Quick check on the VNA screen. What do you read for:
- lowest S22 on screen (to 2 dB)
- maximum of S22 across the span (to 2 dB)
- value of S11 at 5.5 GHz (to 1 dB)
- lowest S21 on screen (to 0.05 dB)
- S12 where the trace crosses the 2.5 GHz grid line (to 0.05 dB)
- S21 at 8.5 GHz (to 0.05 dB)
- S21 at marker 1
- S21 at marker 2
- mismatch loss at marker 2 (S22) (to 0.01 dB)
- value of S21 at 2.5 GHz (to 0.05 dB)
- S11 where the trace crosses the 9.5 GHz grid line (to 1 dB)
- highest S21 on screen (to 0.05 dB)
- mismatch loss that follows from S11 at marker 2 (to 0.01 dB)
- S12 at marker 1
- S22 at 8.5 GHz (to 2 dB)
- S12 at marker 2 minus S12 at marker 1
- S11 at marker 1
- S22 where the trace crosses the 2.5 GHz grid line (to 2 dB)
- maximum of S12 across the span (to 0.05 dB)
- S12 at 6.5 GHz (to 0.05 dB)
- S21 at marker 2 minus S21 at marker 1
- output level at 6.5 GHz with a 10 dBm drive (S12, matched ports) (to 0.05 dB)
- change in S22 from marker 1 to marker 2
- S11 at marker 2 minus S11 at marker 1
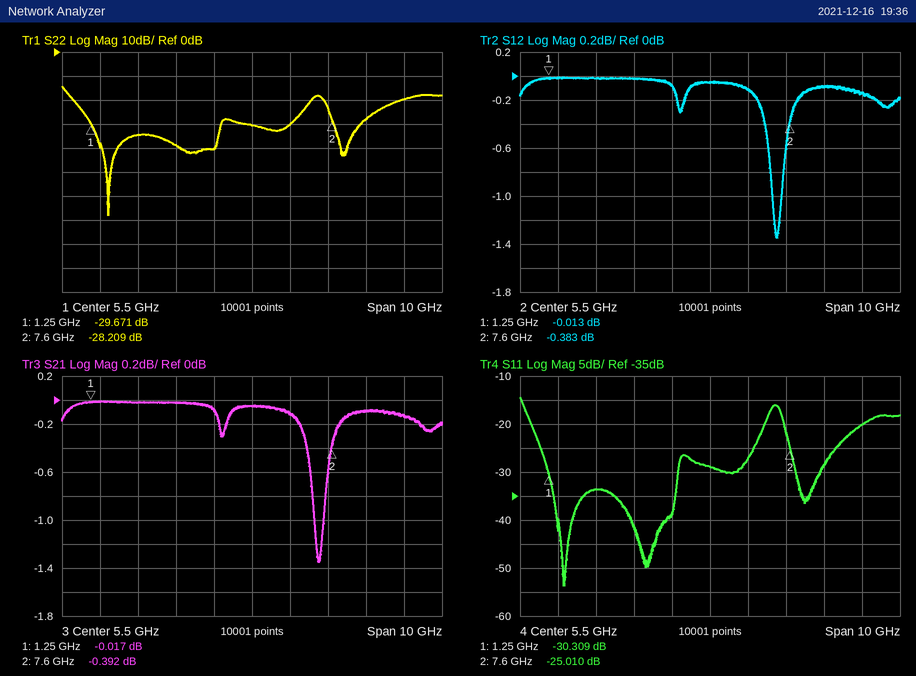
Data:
-68 dB
-14 dB
-29 dB
-1.35 dB
0.00 dB
-0.10 dB
-0.017 dB
-0.392 dB
0.01 dB
0.00 dB
-20 dB
0.00 dB
0.01 dB
-0.013 dB
-28 dB
-0.370 dB
-30.309 dB
-34 dB
0.00 dB
-0.10 dB
-0.375 dB
9.90 dBm
1.462 dB
5.299 dB
